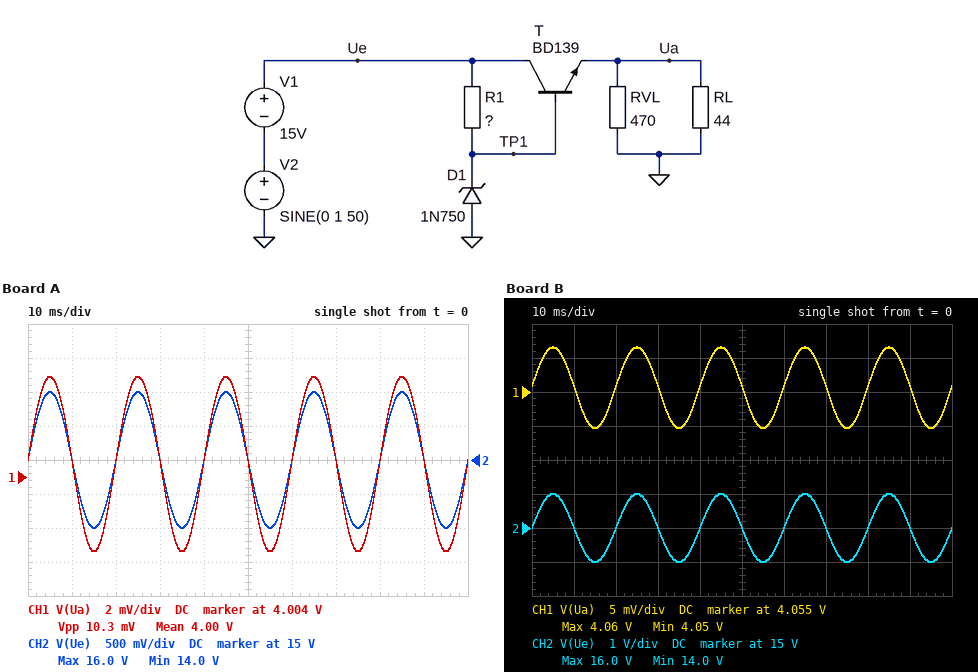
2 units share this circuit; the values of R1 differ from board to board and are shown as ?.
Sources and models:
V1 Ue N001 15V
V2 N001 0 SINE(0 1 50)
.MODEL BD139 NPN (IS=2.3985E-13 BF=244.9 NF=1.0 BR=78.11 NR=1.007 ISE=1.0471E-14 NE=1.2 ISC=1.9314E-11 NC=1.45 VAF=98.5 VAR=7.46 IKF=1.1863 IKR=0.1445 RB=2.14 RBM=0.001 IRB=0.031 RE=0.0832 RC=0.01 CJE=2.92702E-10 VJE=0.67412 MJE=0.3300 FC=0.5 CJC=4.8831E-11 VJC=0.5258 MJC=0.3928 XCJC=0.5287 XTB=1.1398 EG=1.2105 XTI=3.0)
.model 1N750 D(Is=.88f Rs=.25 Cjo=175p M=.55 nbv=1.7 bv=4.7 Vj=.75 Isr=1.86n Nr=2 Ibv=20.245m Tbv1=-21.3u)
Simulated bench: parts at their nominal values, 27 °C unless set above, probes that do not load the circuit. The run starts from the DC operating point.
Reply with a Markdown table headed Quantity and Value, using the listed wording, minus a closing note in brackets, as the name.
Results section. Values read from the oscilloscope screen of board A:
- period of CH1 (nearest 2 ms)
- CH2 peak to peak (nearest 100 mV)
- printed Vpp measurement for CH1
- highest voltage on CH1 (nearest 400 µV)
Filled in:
| Quantity | Value |
|---|---|
| period of CH1 | 20 ms |
| CH2 peak to peak | 2.0 V |
| printed Vpp measurement for CH1 | 10.3 mV |
| highest voltage on CH1 | 4.0100 V |
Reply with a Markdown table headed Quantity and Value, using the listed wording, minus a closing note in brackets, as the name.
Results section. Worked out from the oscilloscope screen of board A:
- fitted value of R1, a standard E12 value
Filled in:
| Quantity | Value |
|---|---|
| fitted value of R1, a standard E12 value | 470 Ω |
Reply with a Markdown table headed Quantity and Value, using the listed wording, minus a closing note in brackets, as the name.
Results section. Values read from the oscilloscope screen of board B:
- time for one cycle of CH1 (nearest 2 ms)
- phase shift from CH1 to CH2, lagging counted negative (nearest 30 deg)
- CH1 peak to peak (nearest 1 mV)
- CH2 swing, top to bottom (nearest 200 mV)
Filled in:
| Quantity | Value |
|---|---|
| time for one cycle of CH1 | 20 ms |
| phase shift from CH1 to CH2, lagging counted negative | 0 deg |
| CH1 peak to peak | 12 mV |
| CH2 swing, top to bottom | 2.0 V |
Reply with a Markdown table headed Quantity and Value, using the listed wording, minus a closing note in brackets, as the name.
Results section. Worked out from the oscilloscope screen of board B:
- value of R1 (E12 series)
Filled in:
| Quantity | Value |
|---|---|
| value of R1 | 180 Ω |
